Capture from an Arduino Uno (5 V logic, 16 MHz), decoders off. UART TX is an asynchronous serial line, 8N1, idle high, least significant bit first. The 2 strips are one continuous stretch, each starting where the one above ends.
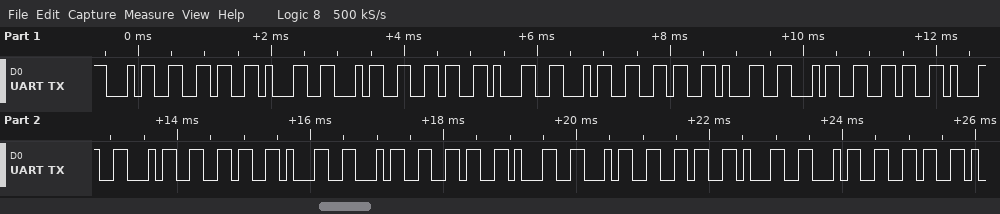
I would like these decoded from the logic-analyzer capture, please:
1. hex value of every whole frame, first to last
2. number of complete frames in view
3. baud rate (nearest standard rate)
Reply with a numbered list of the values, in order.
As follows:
1. 0x34 0x36 0x31 0x34 0x36 0x31 0x34 0x36 0x31 0x34 0x36 0x31 0x34 0x36 0x31 0x34 0x36 0x31 0x34 0x36 0x31 0x34 0x36
2. 23
3. 9600 baud
